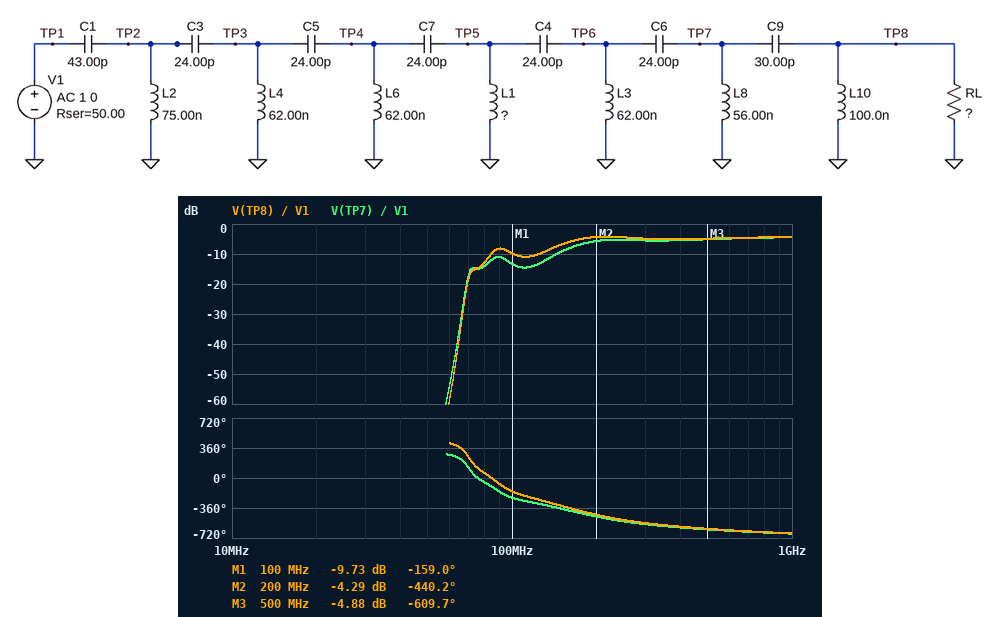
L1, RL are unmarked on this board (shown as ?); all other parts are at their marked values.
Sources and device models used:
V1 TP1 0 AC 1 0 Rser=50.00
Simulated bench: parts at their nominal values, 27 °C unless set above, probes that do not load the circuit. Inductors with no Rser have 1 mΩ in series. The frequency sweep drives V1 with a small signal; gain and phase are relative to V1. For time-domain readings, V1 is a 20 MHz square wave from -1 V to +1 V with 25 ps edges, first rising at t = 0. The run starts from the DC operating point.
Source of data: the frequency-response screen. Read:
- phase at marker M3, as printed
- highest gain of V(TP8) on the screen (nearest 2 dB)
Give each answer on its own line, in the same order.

-609.7 deg
-4 dB
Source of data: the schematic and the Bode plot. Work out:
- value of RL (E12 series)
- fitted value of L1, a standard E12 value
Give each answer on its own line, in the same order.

82 Ω
22 nH
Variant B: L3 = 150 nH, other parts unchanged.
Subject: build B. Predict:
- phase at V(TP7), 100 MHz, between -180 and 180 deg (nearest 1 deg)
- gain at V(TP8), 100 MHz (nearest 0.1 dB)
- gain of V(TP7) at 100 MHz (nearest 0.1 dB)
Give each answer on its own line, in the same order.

100 deg
-15.6 dB
-19.1 dB
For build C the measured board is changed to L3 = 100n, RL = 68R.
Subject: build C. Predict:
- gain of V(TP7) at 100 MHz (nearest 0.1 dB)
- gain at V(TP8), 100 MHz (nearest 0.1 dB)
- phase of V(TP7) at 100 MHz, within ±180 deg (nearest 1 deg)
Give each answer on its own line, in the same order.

-15.9 dB
-13.9 dB
105 deg
